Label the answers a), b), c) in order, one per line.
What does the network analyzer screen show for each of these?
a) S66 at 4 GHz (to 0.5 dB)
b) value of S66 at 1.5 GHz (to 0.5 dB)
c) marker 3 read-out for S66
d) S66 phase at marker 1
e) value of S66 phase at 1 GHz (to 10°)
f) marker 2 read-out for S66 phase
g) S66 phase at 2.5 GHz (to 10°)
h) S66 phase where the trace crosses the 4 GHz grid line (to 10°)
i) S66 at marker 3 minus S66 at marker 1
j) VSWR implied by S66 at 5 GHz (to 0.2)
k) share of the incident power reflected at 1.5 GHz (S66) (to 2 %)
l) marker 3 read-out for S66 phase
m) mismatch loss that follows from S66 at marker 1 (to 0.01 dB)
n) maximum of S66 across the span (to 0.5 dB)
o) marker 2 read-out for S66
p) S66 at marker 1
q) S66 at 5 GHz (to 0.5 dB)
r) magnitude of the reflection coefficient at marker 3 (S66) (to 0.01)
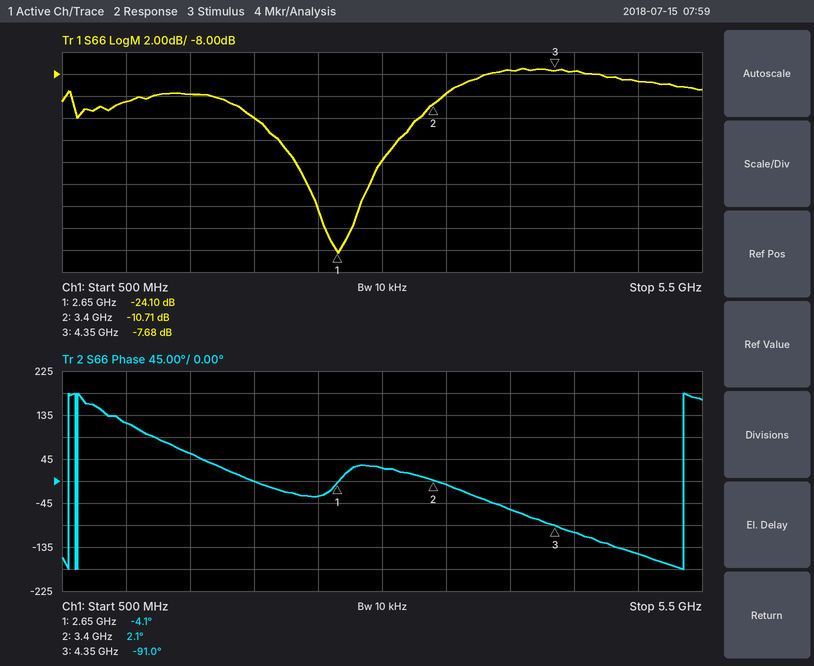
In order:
a) -7.5 dB
b) -10.0 dB
c) -7.68 dB
d) -4.1°
e) 120°
f) 2.1°
g) -30°
h) -60°
i) 16.42 dB
j) 2.2
k) 10 %
l) -91.0°
m) 0.02 dB
n) -7.5 dB
o) -10.71 dB
p) -24.10 dB
q) -8.5 dB
r) 0.41
